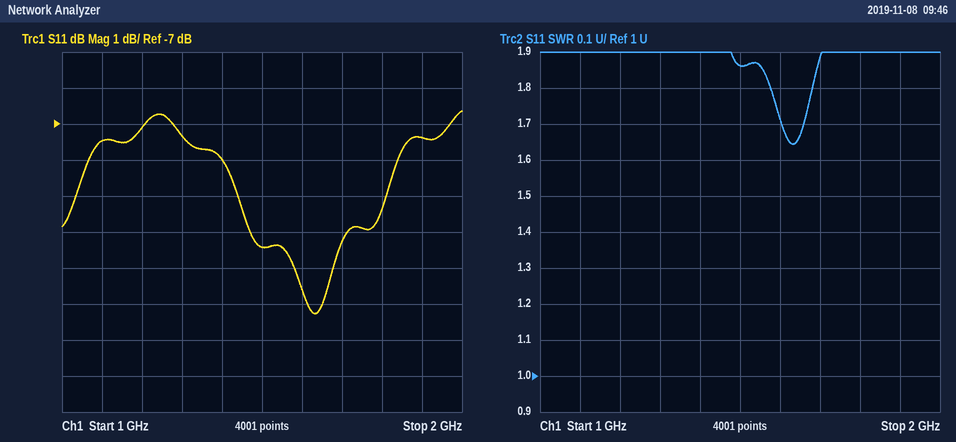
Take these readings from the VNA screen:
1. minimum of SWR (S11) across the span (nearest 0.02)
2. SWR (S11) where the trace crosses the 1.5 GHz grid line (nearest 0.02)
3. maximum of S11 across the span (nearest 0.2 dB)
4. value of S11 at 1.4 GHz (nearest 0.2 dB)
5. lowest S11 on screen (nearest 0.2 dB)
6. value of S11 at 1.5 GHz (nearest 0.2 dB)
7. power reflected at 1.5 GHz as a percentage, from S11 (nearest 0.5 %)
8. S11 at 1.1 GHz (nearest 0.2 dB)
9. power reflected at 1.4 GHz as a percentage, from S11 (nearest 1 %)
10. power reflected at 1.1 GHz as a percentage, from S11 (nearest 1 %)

1.64
1.86
-6.6 dB
-8.0 dB
-12.2 dB
-10.4 dB
9.0 %
-7.4 dB
16 %
18 %
